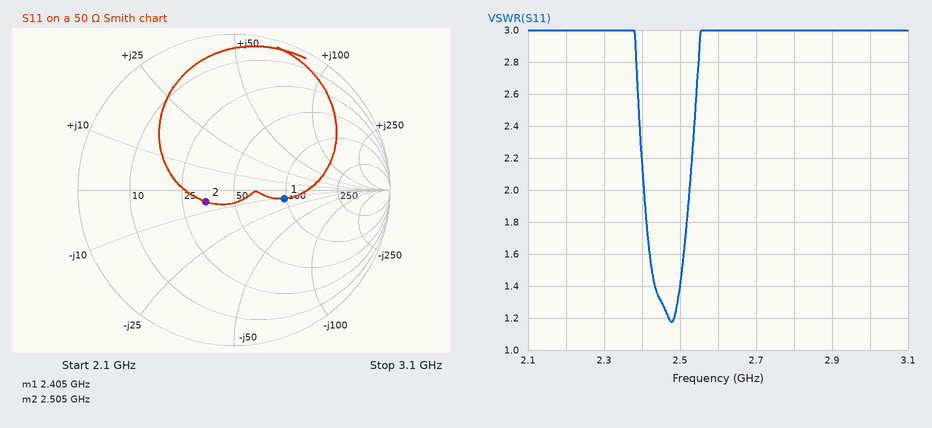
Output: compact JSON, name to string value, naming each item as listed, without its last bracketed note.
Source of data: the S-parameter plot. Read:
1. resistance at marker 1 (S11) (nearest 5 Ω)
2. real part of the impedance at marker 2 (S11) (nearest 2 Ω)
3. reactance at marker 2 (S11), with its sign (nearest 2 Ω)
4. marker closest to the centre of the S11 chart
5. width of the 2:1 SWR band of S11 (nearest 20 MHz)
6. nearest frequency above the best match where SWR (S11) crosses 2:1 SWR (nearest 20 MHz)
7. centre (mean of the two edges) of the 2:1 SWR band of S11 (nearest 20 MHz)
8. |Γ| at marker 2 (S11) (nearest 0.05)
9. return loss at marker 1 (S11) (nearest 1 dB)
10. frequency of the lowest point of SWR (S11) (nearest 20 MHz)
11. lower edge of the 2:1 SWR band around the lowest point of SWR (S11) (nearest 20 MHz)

{"resistance at marker 1 (S11)": "95 Ω", "real part of the impedance at marker 2 (S11)": "34 Ω", "reactance at marker 2 (S11), with its sign": "-6 Ω", "marker closest to the centre of the S11 chart": "marker 2", "width of the 2:1 SWR band of S11": "120 MHz", "nearest frequency above the best match where SWR (S11) crosses 2:1 SWR": "2.52 GHz", "centre (mean of the two edges) of the 2:1 SWR band of S11": "2.46 GHz", "|Γ| at marker 2 (S11)": "0.20", "return loss at marker 1 (S11)": "10 dB", "frequency of the lowest point of SWR (S11)": "2.48 GHz", "lower edge of the 2:1 SWR band around the lowest point of SWR (S11)": "2.40 GHz"}
